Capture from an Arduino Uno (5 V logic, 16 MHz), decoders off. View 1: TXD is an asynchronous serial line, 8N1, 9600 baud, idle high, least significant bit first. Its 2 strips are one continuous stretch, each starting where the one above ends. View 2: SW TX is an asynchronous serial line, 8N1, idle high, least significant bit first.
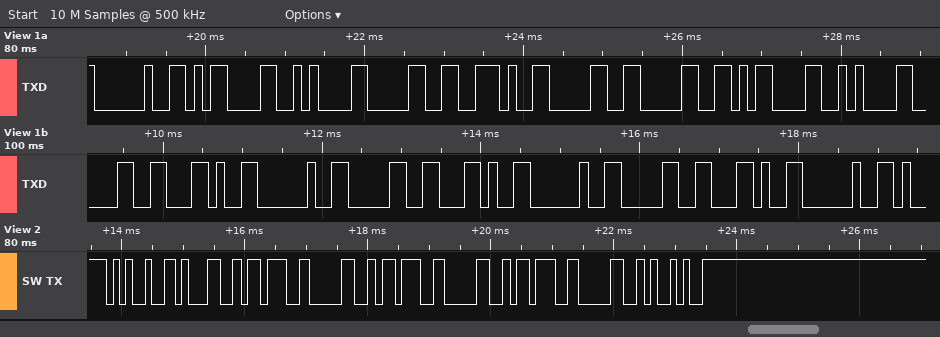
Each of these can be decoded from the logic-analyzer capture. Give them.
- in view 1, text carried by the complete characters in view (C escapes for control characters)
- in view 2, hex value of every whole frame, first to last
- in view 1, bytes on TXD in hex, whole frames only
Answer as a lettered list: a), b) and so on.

a) " \r\n0.00\r\n0, 0, 0, "
b) 25 31 3B 30 3B 30 3B 30 29
c) 0x20 0x0D 0x0A 0x30 0x2E 0x30 0x30 0x0D 0x0A 0x30 0x2C 0x20 0x30 0x2C 0x20 0x30 0x2C 0x20
